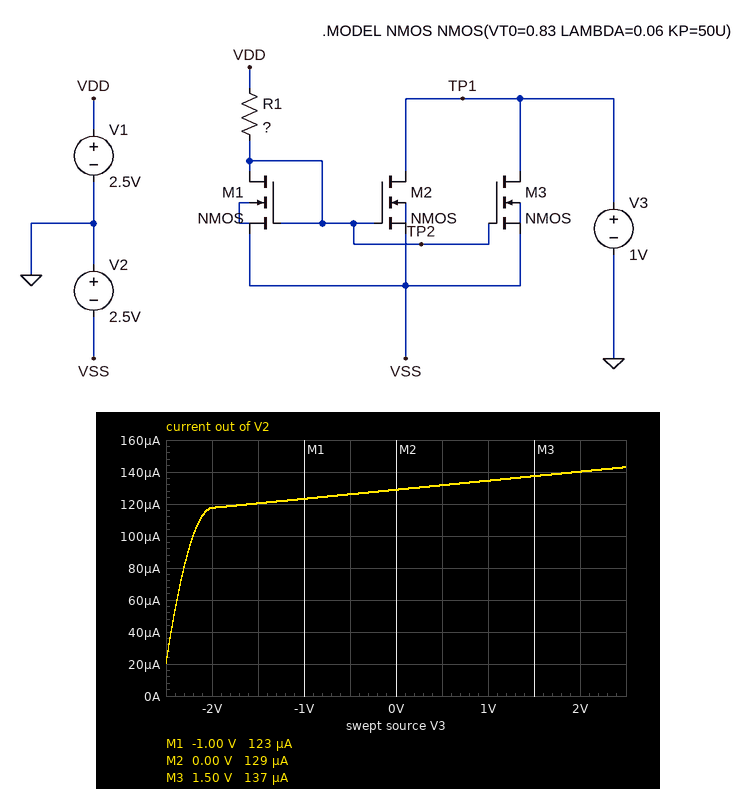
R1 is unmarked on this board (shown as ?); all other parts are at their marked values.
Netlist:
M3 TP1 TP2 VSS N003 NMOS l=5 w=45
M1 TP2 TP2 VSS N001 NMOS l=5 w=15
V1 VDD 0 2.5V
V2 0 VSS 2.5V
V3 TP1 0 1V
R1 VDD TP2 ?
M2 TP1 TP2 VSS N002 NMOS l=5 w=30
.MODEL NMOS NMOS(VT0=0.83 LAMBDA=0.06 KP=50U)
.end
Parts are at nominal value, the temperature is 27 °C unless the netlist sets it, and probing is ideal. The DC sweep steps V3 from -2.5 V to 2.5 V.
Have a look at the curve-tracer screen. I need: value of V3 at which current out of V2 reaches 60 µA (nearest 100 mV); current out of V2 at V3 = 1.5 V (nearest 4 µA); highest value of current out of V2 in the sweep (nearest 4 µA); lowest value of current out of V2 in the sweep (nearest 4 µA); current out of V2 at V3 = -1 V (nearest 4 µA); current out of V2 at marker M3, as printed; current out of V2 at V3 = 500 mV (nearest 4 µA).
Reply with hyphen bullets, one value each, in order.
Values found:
- -2.4 V
- 136 µA
- 144 µA
- 20 µA
- 124 µA
- 137 µA
- 132 µA
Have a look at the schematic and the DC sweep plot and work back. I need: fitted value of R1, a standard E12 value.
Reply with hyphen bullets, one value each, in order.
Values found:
- 180 kΩ
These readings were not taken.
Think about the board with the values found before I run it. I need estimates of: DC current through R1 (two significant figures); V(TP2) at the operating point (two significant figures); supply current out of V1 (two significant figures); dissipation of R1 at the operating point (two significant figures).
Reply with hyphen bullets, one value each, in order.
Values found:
- 20 µA
- -1.2 V
- 20 µA
- 75 µW
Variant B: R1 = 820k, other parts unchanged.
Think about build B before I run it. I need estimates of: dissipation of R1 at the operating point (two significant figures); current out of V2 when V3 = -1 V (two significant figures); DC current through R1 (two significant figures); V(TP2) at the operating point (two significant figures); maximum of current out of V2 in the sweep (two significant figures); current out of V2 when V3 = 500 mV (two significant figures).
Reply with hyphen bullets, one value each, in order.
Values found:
- 19 µW
- 29 µA
- 4.8 µA
- -1.4 V
- 34 µA
- 31 µA
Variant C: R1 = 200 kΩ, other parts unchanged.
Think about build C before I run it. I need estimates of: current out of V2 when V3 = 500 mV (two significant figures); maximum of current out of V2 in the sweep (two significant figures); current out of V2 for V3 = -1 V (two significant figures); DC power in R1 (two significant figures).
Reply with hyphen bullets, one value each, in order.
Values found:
- 120 µA
- 130 µA
- 110 µA
- 68 µW
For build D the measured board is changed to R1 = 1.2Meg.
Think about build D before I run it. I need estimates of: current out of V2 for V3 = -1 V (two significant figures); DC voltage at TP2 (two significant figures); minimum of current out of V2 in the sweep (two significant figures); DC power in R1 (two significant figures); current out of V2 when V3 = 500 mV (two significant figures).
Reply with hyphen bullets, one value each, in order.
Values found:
- 20 µA
- -1.5 V
- 3.3 µA
- 13 µW
- 22 µA
